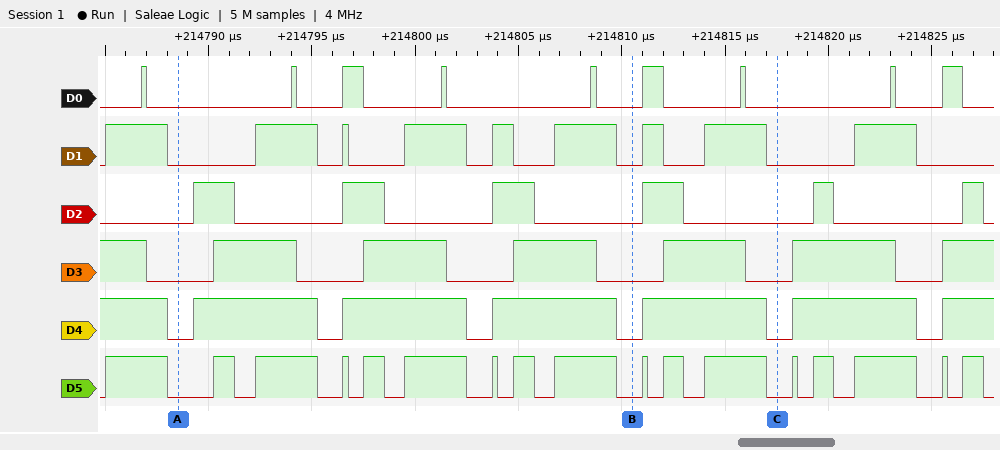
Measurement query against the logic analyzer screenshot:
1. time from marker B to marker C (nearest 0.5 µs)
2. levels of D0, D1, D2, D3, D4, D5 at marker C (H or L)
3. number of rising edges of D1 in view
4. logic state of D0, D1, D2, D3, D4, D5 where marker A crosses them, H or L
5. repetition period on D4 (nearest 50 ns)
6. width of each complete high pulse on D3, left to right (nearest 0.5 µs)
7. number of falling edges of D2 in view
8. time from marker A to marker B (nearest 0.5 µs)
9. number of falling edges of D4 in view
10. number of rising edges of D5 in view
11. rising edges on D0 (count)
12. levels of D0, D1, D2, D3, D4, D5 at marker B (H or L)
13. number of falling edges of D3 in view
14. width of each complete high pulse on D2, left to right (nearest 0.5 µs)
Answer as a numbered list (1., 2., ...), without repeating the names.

1. 7 µs
2. D0=L, D1=L, D2=L, D3=L, D4=L, D5=L
3. 9
4. D0=L, D1=L, D2=L, D3=L, D4=L, D5=L
5. 7250 ns
6. 4 µs, 4 µs, 4 µs, 4 µs, 5 µs
7. 6
8. 22 µs
9. 6
10. 17
11. 9
12. D0=L, D1=L, D2=L, D3=L, D4=L, D5=L
13. 6
14. 2 µs, 2 µs, 2 µs, 2 µs, 1 µs, 1 µs
